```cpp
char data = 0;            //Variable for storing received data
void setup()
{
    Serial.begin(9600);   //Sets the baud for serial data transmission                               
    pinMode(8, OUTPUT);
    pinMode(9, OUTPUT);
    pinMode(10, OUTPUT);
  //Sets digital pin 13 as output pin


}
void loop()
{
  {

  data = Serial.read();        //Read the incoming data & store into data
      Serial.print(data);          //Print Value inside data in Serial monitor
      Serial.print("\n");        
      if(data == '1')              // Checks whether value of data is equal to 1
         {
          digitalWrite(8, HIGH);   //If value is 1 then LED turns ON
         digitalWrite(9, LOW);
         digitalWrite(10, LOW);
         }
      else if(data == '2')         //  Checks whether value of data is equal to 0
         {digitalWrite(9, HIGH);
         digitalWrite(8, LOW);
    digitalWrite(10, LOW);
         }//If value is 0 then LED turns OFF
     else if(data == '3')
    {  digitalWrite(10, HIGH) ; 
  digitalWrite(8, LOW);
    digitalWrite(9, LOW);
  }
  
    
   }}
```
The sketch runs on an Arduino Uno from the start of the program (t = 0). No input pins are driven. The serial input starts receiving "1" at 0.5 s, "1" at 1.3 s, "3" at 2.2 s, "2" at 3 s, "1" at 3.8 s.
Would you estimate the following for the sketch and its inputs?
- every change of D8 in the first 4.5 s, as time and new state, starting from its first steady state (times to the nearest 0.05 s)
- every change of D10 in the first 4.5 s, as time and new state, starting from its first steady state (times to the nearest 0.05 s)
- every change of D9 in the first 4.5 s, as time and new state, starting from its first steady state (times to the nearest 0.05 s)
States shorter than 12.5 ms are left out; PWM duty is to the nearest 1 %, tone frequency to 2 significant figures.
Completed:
0 s low; 0.5 s high; 2.2 s low; 3.8 s high
0 s low; 2.2 s high; 3 s low
0 s low; 3 s high; 3.8 s low
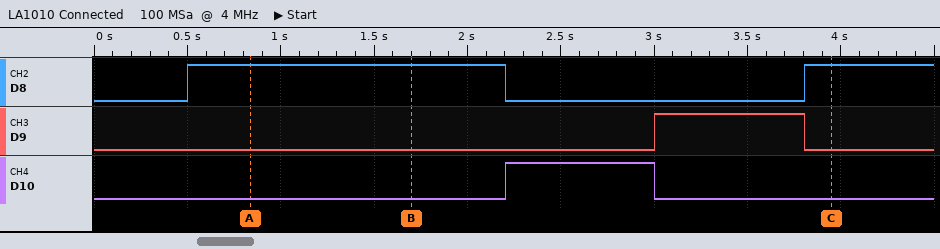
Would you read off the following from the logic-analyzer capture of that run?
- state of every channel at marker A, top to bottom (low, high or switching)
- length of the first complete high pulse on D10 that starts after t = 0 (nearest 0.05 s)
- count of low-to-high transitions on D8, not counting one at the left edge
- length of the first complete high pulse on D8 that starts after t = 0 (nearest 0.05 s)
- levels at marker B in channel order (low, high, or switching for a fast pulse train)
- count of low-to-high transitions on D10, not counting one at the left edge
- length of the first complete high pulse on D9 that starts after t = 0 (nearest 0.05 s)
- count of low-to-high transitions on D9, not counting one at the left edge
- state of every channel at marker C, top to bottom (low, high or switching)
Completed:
D8 high, D9 low, D10 low
0.80 s
2
1.70 s
D8 high, D9 low, D10 low
1
0.80 s
1
D8 high, D9 low, D10 low
